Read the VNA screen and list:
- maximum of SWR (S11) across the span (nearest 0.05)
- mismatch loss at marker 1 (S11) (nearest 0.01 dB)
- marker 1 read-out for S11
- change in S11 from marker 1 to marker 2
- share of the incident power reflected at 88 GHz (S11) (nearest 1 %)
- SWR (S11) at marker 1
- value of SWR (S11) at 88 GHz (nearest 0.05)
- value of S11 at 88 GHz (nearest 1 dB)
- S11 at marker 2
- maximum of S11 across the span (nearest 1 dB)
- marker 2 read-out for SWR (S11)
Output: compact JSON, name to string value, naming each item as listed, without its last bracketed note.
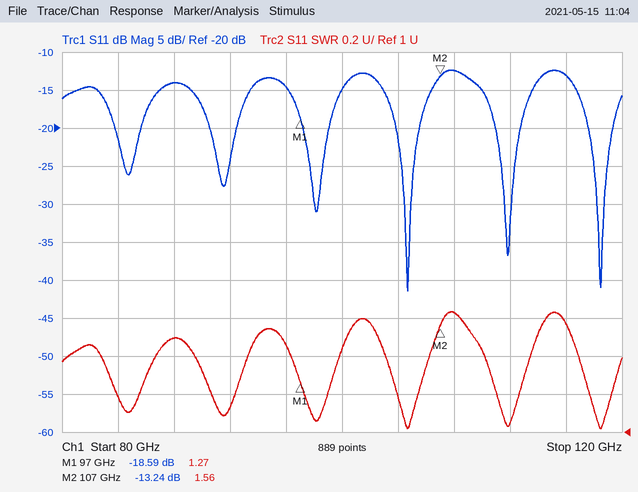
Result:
{"maximum of SWR (S11) across the span": "1.65", "mismatch loss at marker 1 (S11)": "0.06 dB", "marker 1 read-out for S11": "-18.59 dB", "change in S11 from marker 1 to marker 2": "5.35 dB", "share of the incident power reflected at 88 GHz (S11)": "4 %", "SWR (S11) at marker 1": "1.27", "value of SWR (S11) at 88 GHz": "1.50", "value of S11 at 88 GHz": "-14 dB", "S11 at marker 2": "-13.24 dB", "maximum of S11 across the span": "-12 dB", "marker 2 read-out for SWR": "1.56"}
